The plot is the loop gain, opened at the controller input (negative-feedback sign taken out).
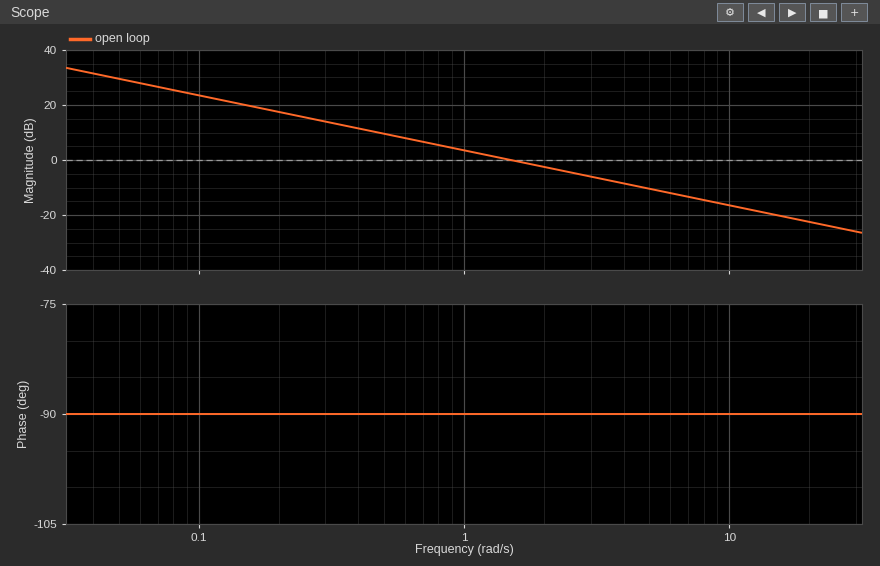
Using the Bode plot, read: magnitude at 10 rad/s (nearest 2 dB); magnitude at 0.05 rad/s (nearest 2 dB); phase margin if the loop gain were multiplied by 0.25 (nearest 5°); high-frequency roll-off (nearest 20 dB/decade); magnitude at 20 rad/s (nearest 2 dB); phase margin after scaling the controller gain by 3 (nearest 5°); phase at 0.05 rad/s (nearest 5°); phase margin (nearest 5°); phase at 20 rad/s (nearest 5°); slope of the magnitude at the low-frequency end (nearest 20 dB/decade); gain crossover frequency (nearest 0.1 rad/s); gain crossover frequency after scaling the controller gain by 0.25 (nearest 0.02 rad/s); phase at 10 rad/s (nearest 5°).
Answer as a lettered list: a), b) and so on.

a) -16 dB
b) 30 dB
c) 90°
d) -20 dB/decade
e) -22 dB
f) 90°
g) -90°
h) 90°
i) -90°
j) -20 dB/decade
k) 1.5 rad/s
l) 0.38 rad/s
m) -90°
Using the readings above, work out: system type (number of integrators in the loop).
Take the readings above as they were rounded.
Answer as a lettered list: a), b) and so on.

a) 1
